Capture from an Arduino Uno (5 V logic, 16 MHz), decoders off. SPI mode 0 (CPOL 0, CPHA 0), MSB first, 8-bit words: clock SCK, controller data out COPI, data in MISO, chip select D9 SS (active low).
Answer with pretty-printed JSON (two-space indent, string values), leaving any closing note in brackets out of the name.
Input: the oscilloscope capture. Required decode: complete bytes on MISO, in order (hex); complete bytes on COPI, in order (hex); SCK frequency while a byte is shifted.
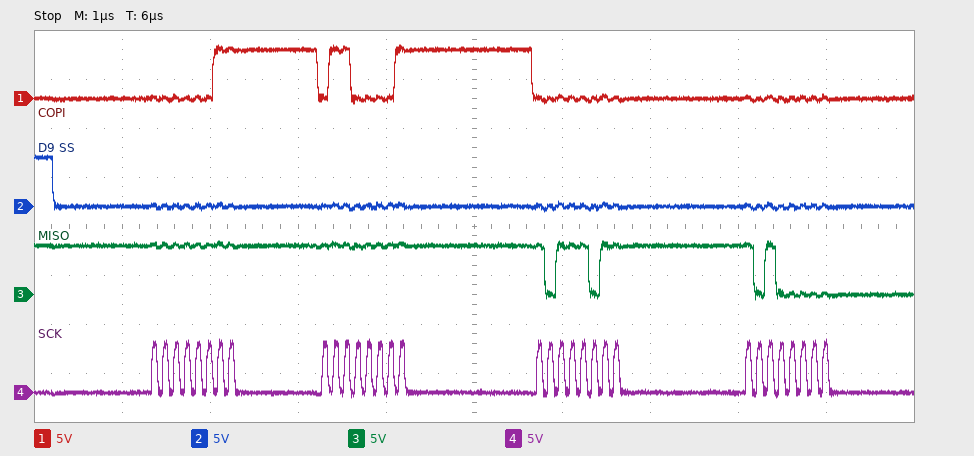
{
  "complete bytes on MISO, in order": "FF FF BB A0",
  "complete bytes on COPI, in order": "03 61 00 00",
  "SCK frequency while a byte is shifted": "8 MHz"
}
